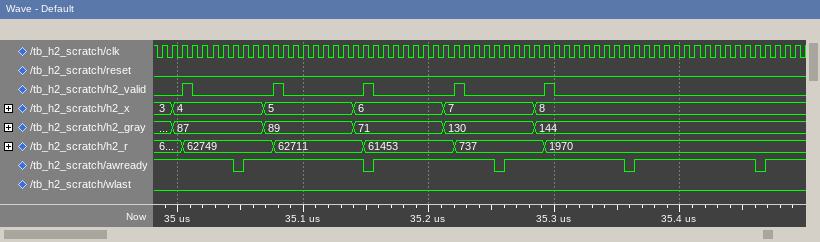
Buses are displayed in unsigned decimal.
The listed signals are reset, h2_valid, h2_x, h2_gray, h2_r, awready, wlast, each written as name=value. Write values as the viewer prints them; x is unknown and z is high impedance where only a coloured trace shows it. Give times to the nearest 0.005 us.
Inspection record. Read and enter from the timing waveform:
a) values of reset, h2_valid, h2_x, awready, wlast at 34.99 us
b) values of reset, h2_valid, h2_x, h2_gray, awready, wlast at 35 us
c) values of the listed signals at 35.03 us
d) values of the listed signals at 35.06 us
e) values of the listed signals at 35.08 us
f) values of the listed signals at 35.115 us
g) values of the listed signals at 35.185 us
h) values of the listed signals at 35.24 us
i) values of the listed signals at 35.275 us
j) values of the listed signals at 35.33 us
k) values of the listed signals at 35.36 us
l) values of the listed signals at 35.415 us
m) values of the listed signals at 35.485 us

reset=0, h2_valid=0, h2_x=3, awready=1, wlast=0
reset=0, h2_valid=0, h2_x=4, h2_gray=87, awready=1, wlast=0
reset=0, h2_valid=0, h2_x=4, h2_gray=87, h2_r=62749, awready=1, wlast=0
reset=0, h2_valid=0, h2_x=4, h2_gray=87, h2_r=62749, awready=1, wlast=0
reset=0, h2_valid=1, h2_x=5, h2_gray=89, h2_r=62711, awready=1, wlast=0
reset=0, h2_valid=0, h2_x=5, h2_gray=89, h2_r=62711, awready=1, wlast=0
reset=0, h2_valid=0, h2_x=6, h2_gray=71, h2_r=61453, awready=1, wlast=0
reset=0, h2_valid=0, h2_x=7, h2_gray=130, h2_r=737, awready=1, wlast=0
reset=0, h2_valid=0, h2_x=7, h2_gray=130, h2_r=737, awready=1, wlast=0
reset=0, h2_valid=0, h2_x=8, h2_gray=144, h2_r=1970, awready=1, wlast=0
reset=0, h2_valid=0, h2_x=8, h2_gray=144, h2_r=1970, awready=0, wlast=0
reset=0, h2_valid=0, h2_x=8, h2_gray=144, h2_r=1970, awready=1, wlast=0
reset=0, h2_valid=0, h2_x=8, h2_gray=144, h2_r=1970, awready=1, wlast=0
